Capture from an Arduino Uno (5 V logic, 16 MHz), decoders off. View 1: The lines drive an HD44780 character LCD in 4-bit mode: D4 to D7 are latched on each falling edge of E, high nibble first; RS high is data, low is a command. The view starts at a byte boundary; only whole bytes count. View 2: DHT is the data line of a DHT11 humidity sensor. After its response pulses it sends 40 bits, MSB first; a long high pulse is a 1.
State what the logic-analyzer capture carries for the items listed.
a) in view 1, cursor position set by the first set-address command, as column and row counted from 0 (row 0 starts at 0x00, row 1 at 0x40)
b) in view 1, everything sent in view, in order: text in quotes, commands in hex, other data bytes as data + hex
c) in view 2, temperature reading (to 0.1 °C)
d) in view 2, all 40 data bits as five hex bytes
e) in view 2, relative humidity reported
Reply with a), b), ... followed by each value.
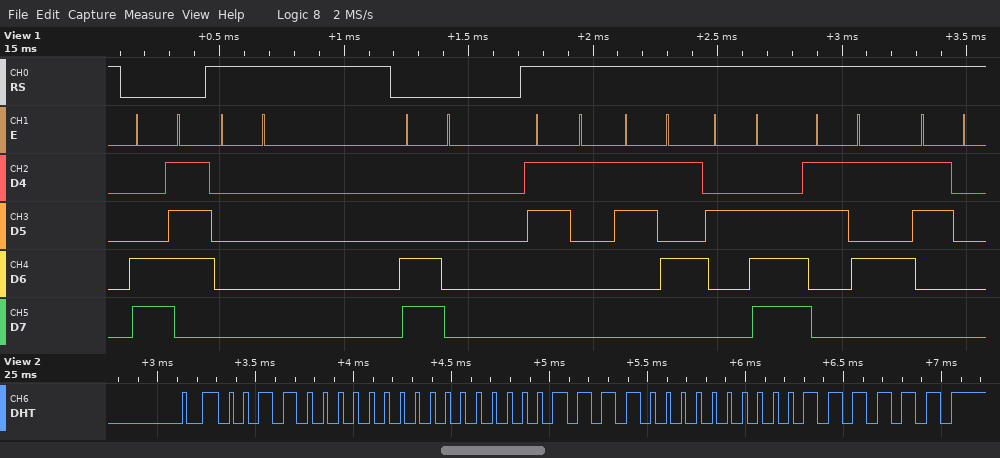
a) column 7, row 1
b) 0xC7 data 00 0xC0 "15.50"
c) 15.0 °C
d) 30 00 0F 00 3F
e) 48 %
